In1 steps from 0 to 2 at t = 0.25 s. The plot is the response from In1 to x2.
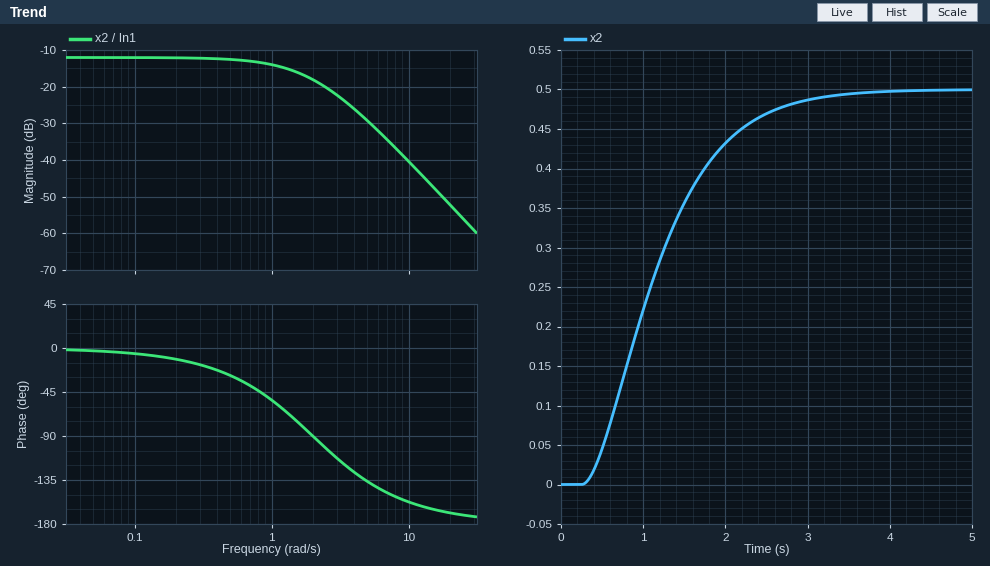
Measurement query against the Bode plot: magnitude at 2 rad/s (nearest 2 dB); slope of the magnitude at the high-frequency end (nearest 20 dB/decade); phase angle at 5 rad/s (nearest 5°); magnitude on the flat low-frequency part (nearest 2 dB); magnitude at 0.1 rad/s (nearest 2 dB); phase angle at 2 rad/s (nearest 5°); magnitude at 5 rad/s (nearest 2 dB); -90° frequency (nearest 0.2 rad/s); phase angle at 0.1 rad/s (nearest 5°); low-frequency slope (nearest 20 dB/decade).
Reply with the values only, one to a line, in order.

-18 dB
-40 dB/decade
-135°
-12 dB
-12 dB
-90°
-30 dB
2.0 rad/s
-5°
0 dB/decade
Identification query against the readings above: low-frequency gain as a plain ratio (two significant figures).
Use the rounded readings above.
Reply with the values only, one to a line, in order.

0.25
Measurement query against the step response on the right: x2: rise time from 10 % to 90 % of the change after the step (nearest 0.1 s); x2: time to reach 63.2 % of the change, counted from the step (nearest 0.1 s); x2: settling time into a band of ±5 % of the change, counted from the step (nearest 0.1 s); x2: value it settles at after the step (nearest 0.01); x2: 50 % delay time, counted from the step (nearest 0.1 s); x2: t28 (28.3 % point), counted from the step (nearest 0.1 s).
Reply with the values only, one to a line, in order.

1.7 s
1.1 s
2.4 s
0.50
0.8 s
0.5 s
